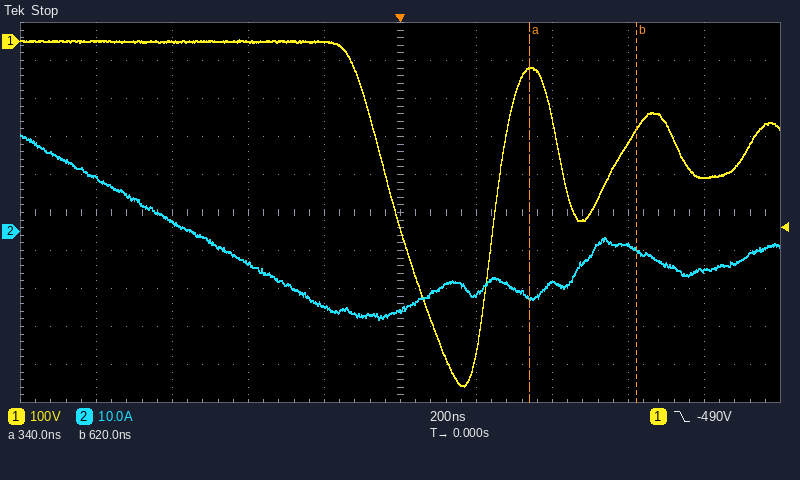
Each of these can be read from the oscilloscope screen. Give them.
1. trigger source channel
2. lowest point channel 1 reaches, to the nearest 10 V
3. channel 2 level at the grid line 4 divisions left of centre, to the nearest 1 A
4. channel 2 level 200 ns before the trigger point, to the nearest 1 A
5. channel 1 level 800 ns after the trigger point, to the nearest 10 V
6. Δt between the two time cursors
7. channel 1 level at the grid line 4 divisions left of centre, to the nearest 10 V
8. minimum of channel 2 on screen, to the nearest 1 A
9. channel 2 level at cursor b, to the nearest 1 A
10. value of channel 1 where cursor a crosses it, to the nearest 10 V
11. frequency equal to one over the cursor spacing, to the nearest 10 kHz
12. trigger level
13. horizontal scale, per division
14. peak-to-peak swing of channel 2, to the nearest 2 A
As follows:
channel 1
-910 V
14 A
-20 A
-360 V
280 ns
0 V
-23 A
-5 A
-70 V
3.57 MHz
-490 V
200 ns
48 A
